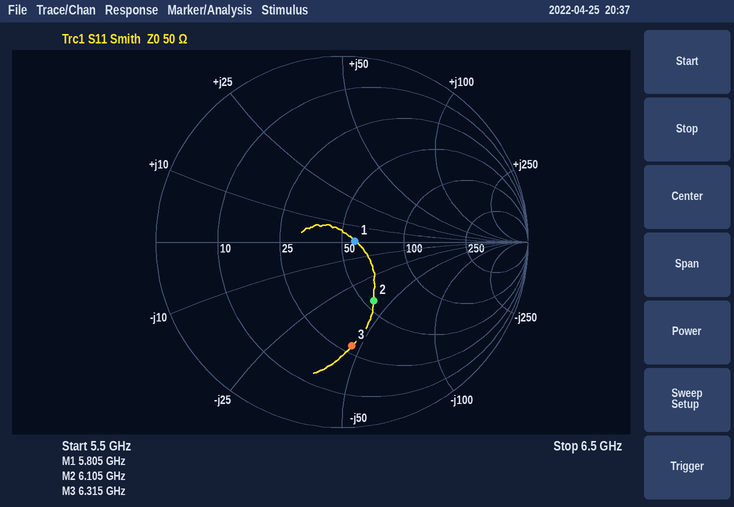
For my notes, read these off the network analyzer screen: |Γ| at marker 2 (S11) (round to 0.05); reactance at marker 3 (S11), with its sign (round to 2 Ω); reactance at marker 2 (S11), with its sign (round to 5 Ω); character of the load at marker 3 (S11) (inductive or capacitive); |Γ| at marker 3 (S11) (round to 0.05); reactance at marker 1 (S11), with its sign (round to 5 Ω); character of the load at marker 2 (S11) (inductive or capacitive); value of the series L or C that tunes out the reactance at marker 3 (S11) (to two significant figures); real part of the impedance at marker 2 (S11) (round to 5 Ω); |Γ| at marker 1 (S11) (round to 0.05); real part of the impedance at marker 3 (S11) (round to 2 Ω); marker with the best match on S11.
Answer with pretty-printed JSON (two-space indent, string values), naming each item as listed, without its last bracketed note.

{
  "|Γ| at marker 2 (S11)": "0.35",
  "reactance at marker 3 (S11), with its sign": "-46 Ω",
  "reactance at marker 2 (S11), with its sign": "-40 Ω",
  "character of the load at marker 3 (S11)": "capacitive",
  "|Γ| at marker 3 (S11)": "0.55",
  "reactance at marker 1 (S11), with its sign": "0 Ω",
  "character of the load at marker 2 (S11)": "capacitive",
  "value of the series L or C that tunes out the reactance at marker 3 (S11)": "1.2 nH",
  "real part of the impedance at marker 2 (S11)": "55 Ω",
  "|Γ| at marker 1 (S11)": "0.05",
  "real part of the impedance at marker 3 (S11)": "28 Ω",
  "marker with the best match on S11": "marker 1"
}
